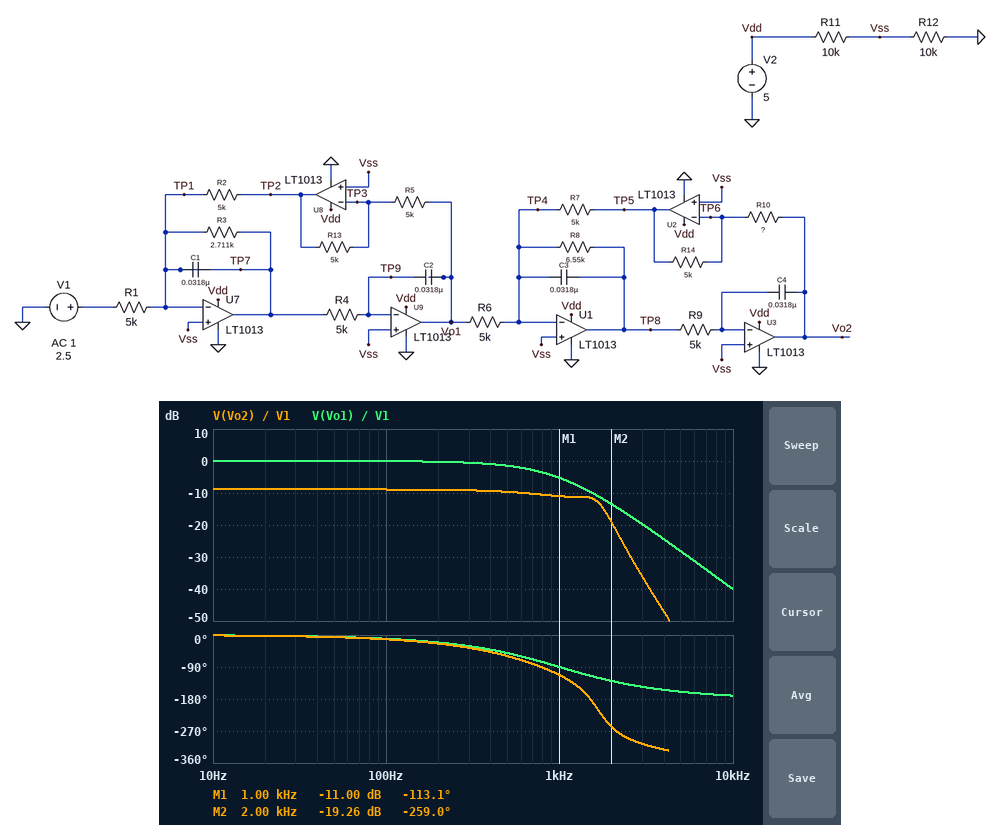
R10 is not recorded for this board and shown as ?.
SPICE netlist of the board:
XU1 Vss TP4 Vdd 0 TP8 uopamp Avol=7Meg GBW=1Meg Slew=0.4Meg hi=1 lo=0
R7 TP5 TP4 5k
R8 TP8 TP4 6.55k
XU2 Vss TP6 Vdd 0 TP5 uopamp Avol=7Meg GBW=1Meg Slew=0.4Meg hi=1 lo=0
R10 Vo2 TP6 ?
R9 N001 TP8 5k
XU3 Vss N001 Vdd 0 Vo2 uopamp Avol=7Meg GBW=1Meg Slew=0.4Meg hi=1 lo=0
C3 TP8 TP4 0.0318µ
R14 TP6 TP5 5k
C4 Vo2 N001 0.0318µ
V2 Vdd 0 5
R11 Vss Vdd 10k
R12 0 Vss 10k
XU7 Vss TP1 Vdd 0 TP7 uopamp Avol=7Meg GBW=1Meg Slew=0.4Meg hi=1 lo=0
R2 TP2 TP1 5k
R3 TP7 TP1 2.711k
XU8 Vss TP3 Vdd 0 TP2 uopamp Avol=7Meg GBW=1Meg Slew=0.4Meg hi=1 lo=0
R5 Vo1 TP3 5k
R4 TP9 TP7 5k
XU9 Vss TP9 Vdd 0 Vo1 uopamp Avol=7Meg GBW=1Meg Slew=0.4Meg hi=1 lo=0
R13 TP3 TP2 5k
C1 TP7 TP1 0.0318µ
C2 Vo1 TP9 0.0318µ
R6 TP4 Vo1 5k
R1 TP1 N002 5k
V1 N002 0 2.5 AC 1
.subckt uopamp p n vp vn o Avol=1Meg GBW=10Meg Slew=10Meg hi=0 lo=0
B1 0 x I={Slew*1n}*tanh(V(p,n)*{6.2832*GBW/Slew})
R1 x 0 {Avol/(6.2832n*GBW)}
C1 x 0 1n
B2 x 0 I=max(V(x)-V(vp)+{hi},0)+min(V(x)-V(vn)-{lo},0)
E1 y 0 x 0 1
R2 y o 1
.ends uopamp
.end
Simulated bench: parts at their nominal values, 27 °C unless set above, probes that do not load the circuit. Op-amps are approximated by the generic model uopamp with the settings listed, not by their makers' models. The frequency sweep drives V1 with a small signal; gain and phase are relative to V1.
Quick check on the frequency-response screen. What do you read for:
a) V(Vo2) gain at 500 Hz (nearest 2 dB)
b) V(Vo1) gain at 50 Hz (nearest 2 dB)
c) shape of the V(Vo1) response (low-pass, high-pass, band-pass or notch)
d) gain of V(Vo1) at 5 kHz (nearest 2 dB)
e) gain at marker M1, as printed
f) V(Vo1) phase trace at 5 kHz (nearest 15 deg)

-10 dB
0 dB
low-pass
-28 dB
-11.00 dB
-165 deg
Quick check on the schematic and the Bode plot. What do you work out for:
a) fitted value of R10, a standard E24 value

1.8 kΩ
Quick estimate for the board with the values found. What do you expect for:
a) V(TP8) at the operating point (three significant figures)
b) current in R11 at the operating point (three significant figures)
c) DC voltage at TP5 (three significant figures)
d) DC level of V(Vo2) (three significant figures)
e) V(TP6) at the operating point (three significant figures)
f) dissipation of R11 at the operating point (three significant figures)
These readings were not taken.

2.50 V
250 µA
2.50 V
2.50 V
2.50 V
625 µW
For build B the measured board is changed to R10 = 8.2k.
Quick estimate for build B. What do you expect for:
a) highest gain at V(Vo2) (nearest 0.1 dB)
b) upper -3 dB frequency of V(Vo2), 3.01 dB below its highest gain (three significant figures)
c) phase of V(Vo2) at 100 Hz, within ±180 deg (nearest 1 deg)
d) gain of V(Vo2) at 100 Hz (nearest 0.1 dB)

4.4 dB
764 Hz
-18 deg
4.3 dB
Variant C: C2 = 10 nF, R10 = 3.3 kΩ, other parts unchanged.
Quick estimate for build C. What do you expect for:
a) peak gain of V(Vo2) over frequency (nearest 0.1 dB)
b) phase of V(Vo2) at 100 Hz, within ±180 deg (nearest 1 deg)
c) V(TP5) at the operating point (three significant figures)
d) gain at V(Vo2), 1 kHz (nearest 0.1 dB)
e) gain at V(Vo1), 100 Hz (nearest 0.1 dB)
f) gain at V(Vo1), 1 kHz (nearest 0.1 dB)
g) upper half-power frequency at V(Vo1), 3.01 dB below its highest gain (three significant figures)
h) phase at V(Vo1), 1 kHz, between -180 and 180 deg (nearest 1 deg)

2.1 dB
-6 deg
2.50 V
1.7 dB
0 dB
1.0 dB
2.07 kHz
-40 deg
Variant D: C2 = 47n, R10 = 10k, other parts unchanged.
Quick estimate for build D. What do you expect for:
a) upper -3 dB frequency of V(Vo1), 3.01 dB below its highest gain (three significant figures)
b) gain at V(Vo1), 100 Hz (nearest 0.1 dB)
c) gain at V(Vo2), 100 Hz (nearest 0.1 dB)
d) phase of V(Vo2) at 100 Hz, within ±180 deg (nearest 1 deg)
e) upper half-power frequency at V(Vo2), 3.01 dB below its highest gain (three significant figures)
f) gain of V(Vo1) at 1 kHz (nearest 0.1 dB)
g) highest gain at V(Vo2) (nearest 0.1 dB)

452 Hz
-0.2 dB
5.9 dB
-24 deg
523 Hz
-8.8 dB
6.0 dB
